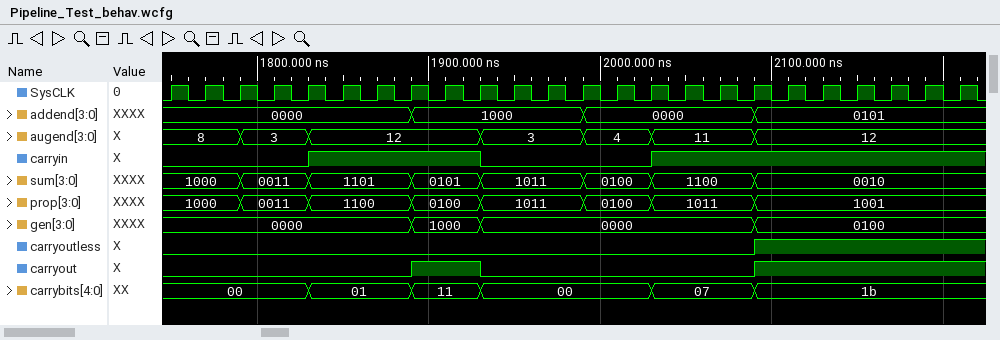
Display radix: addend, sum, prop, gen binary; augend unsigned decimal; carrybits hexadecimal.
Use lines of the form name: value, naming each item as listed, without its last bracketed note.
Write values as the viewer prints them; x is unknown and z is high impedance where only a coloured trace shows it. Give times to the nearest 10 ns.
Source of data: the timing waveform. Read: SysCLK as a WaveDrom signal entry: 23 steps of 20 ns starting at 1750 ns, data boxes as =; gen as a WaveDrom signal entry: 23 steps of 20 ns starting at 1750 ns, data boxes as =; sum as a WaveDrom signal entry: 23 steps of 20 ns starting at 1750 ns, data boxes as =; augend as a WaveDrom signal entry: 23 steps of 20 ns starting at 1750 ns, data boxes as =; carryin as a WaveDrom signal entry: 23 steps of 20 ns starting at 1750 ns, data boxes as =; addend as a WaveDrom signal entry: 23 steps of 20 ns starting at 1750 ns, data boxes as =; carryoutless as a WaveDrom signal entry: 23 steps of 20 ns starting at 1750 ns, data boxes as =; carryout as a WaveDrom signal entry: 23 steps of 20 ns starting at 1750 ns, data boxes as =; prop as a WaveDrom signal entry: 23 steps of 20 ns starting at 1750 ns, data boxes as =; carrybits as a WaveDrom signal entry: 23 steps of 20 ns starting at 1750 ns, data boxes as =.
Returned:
SysCLK as a WaveDrom signal entry: 23 steps of 20 ns starting at 1750 ns, data boxes as =: {name: 'SysCLK', wave: 'p......................'}
gen as a WaveDrom signal entry: 23 steps of 20 ns starting at 1750 ns, data boxes as =: {name: 'gen', wave: '=......=.=.......=.....', data: '0000 1000 0000 0100'}
sum as a WaveDrom signal entry: 23 steps of 20 ns starting at 1750 ns, data boxes as =: {name: 'sum', wave: '=.=.=..=.=..=.=..=.....', data: '1000 0011 1101 0101 1011 0100 1100 0010'}
augend as a WaveDrom signal entry: 23 steps of 20 ns starting at 1750 ns, data boxes as =: {name: 'augend', wave: '=.=.=....=..=.=..=.....', data: '8 3 12 3 4 11 12'}
carryin as a WaveDrom signal entry: 23 steps of 20 ns starting at 1750 ns, data boxes as =: {name: 'carryin', wave: '0...1....0....1........'}
addend as a WaveDrom signal entry: 23 steps of 20 ns starting at 1750 ns, data boxes as =: {name: 'addend', wave: '=......=....=....=.....', data: '0000 1000 0000 0101'}
carryoutless as a WaveDrom signal entry: 23 steps of 20 ns starting at 1750 ns, data boxes as =: {name: 'carryoutless', wave: '0................1.....'}
carryout as a WaveDrom signal entry: 23 steps of 20 ns starting at 1750 ns, data boxes as =: {name: 'carryout', wave: '0......1.0.......1.....'}
prop as a WaveDrom signal entry: 23 steps of 20 ns starting at 1750 ns, data boxes as =: {name: 'prop', wave: '=.=.=..=.=..=.=..=.....', data: '1000 0011 1100 0100 1011 0100 1011 1001'}
carrybits as a WaveDrom signal entry: 23 steps of 20 ns starting at 1750 ns, data boxes as =: {name: 'carrybits', wave: '=...=..=.=....=..=.....', data: '00 01 11 00 07 1b'}
